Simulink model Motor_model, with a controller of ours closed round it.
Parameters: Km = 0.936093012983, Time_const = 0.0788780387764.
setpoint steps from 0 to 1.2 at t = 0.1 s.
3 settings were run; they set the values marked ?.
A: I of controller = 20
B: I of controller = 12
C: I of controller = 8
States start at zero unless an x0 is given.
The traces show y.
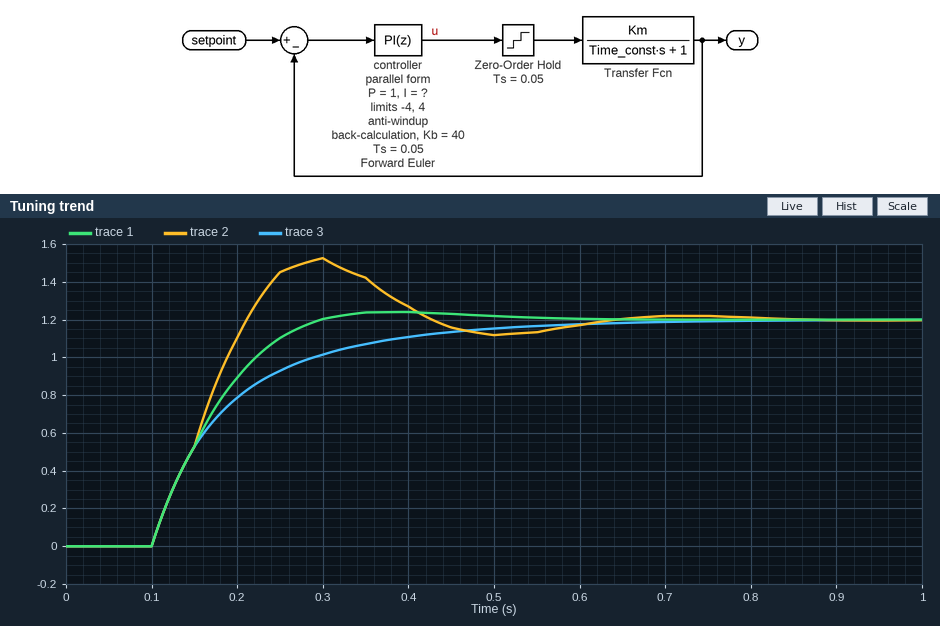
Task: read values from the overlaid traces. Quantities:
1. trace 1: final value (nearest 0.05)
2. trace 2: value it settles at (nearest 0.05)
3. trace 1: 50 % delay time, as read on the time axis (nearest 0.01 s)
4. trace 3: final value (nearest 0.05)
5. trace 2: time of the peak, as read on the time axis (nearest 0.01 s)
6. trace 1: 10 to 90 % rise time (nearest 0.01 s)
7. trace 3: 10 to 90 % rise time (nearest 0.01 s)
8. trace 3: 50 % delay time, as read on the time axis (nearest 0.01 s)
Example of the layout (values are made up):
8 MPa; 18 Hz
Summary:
1.20; 1.20; 0.16 s; 1.20; 0.30 s; 0.13 s; 0.25 s; 0.16 s
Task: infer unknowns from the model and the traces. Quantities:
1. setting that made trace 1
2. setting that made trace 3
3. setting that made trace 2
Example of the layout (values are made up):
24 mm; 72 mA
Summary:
B; C; A
